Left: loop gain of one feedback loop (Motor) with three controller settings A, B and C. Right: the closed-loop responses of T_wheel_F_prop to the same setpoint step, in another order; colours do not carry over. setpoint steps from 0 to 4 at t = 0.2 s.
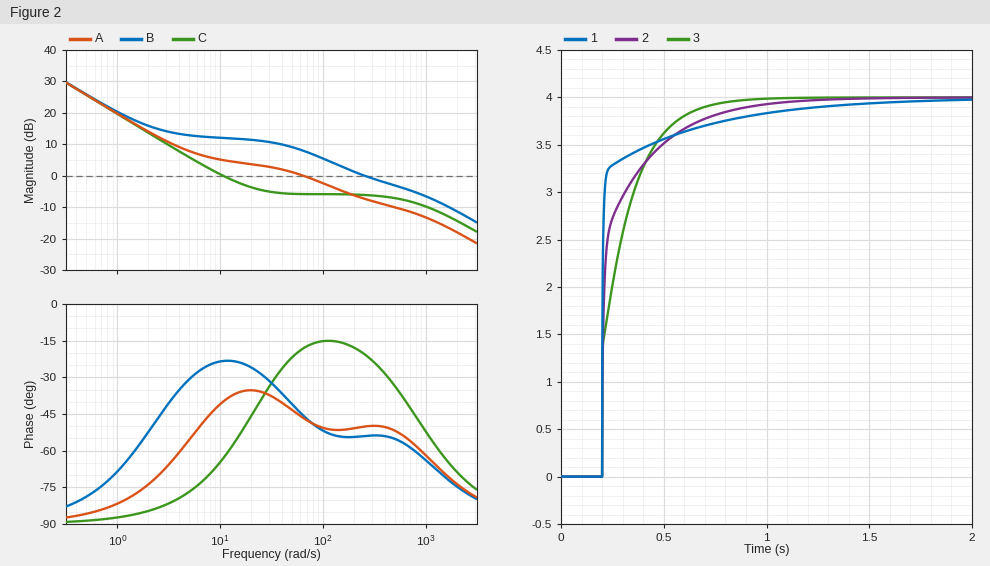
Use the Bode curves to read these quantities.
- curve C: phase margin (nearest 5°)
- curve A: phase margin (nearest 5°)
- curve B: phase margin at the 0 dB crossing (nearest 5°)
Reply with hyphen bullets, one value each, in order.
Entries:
- 115°
- 135°
- 125°
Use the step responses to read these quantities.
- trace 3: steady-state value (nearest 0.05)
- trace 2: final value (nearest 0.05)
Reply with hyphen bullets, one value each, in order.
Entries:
- 4.00
- 4.00
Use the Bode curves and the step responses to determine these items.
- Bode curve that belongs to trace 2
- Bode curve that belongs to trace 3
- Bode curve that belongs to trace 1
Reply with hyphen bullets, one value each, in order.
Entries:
- A
- C
- B
